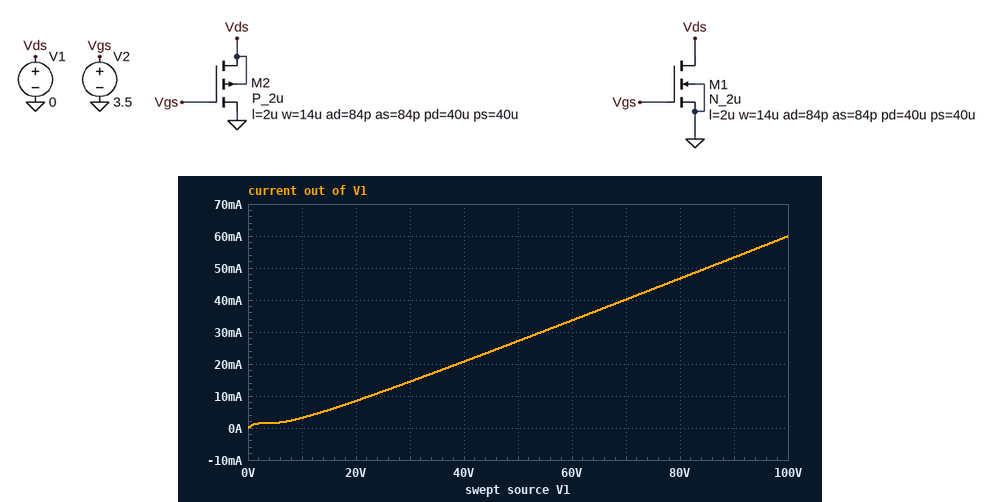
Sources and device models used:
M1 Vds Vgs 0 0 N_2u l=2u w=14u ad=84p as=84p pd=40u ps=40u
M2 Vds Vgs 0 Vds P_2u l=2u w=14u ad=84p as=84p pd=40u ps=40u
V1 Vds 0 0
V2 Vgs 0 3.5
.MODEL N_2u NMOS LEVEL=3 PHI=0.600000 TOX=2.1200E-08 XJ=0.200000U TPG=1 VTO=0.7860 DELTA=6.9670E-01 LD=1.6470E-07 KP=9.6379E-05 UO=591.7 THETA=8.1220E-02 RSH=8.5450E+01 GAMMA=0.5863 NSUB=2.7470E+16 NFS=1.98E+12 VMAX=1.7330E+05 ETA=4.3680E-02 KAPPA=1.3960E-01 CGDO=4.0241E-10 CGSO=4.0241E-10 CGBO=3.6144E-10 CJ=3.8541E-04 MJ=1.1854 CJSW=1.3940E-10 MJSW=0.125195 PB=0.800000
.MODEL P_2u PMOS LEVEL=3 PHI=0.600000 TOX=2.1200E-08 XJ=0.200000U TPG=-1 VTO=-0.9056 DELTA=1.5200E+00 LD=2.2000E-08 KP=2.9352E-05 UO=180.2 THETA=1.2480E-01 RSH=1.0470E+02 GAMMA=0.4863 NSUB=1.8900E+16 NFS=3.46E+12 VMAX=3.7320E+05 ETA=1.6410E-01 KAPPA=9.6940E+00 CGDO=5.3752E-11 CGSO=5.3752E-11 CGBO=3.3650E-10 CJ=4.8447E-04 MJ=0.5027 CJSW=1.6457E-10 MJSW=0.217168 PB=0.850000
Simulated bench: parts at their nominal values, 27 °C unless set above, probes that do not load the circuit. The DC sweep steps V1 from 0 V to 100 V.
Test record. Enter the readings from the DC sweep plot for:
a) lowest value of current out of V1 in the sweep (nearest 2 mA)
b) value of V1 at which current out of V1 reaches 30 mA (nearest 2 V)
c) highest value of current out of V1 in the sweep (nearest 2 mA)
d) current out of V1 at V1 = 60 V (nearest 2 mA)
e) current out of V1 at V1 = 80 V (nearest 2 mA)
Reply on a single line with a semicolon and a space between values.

0 A; 54 V; 60 mA; 34 mA; 46 mA
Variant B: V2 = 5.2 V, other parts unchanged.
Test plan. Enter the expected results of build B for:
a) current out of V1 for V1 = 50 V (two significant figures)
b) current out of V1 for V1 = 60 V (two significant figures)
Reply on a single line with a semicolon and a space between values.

28 mA; 35 mA
